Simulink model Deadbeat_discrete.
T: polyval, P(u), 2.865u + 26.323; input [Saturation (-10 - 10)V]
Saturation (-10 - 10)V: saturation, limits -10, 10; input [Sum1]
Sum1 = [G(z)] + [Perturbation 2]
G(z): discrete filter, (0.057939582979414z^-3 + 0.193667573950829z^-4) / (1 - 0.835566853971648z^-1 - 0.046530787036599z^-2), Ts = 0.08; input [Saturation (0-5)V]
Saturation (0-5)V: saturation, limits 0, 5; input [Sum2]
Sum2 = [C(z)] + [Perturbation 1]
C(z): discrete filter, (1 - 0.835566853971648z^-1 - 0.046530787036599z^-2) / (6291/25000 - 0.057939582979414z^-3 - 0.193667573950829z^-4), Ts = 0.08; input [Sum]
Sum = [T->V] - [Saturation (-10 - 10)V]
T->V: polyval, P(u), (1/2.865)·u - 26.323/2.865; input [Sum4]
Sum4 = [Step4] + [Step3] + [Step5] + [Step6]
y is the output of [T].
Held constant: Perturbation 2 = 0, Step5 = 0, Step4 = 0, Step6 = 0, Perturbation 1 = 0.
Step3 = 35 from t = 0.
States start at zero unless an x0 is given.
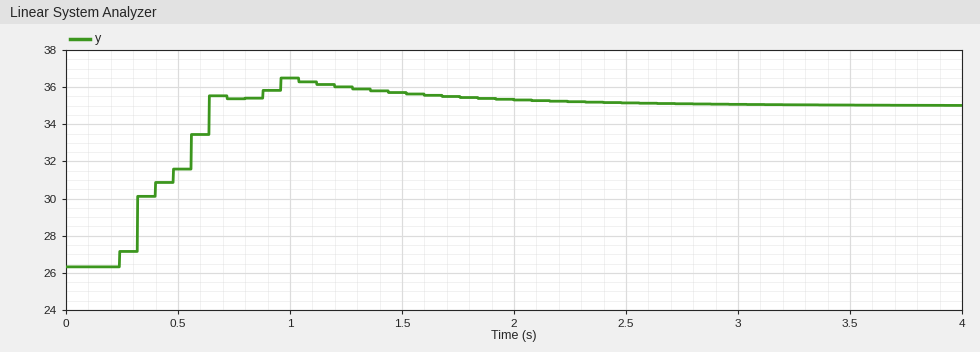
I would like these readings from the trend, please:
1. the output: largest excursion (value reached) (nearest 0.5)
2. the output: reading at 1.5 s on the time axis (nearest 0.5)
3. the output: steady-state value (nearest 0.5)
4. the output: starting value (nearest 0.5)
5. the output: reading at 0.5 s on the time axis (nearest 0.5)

36.5
35.5
35.0
26.5
31.5
